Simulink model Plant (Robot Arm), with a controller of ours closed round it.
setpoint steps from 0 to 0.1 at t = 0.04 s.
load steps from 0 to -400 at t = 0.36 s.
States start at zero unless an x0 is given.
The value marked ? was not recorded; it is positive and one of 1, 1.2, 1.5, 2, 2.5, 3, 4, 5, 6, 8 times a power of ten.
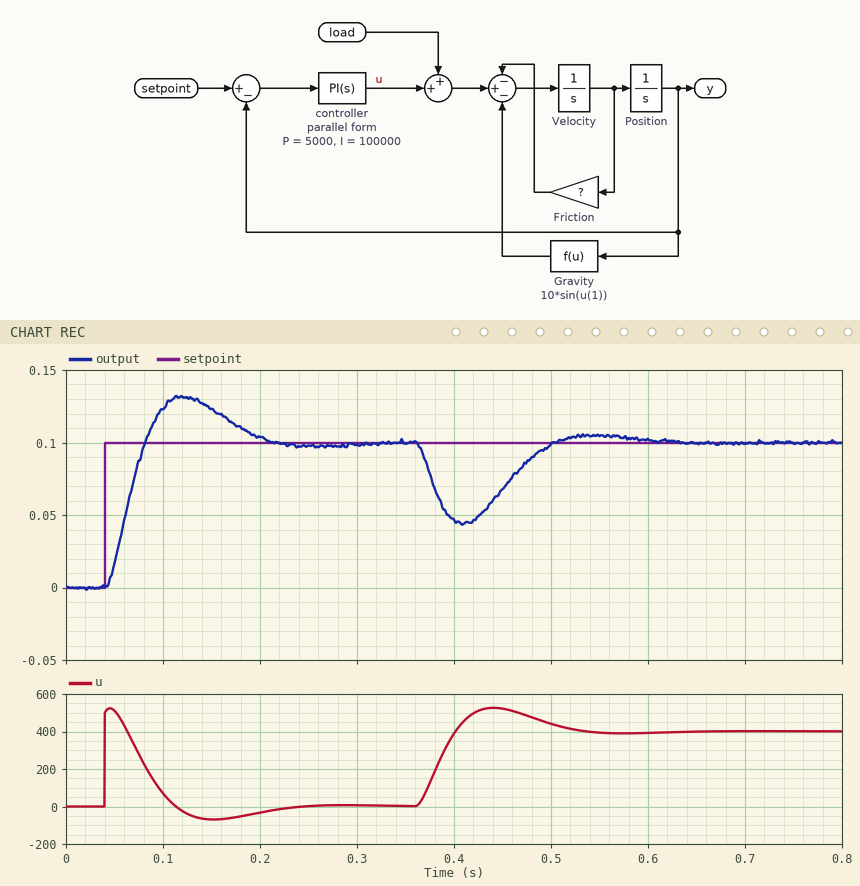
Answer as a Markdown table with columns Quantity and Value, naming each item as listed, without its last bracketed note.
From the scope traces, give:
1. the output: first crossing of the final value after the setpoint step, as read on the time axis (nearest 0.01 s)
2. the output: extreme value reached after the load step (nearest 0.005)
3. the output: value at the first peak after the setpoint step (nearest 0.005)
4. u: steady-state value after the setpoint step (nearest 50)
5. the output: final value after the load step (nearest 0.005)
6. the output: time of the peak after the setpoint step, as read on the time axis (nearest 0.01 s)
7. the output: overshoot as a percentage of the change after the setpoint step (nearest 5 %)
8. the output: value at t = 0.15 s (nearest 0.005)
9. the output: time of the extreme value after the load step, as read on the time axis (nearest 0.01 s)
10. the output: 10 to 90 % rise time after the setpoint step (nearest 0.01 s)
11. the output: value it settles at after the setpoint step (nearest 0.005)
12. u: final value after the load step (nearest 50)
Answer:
| Quantity | Value |
|---|---|
| the output: first crossing of the final value after the setpoint step, as read on the time axis | 0.08 s |
| the output: extreme value reached after the load step | 0.045 |
| the output: value at the first peak after the setpoint step | 0.130 |
| u: steady-state value after the setpoint step | 0 |
| the output: final value after the load step | 0.100 |
| the output: time of the peak after the setpoint step, as read on the time axis | 0.12 s |
| the output: overshoot as a percentage of the change after the setpoint step | 30 % |
| the output: value at t = 0.15 s | 0.125 |
| the output: time of the extreme value after the load step, as read on the time axis | 0.41 s |
| the output: 10 to 90 % rise time after the setpoint step | 0.03 s |
| the output: value it settles at after the setpoint step | 0.100 |
| u: final value after the load step | 400 |
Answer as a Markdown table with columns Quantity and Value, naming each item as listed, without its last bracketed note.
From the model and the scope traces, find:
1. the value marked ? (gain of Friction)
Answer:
| Quantity | Value |
|---|---|
| the value marked ? | 150 |
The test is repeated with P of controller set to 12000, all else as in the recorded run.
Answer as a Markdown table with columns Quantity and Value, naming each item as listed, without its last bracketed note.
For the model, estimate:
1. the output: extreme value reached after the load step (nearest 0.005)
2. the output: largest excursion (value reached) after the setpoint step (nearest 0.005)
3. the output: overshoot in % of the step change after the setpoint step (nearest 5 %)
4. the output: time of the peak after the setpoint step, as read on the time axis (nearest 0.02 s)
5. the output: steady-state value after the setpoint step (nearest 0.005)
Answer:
| Quantity | Value |
|---|---|
| the output: extreme value reached after the load step | 0.070 |
| the output: largest excursion (value reached) after the setpoint step | 0.115 |
| the output: overshoot in % of the step change after the setpoint step | 15 % |
| the output: time of the peak after the setpoint step, as read on the time axis | 0.08 s |
| the output: steady-state value after the setpoint step | 0.100 |
